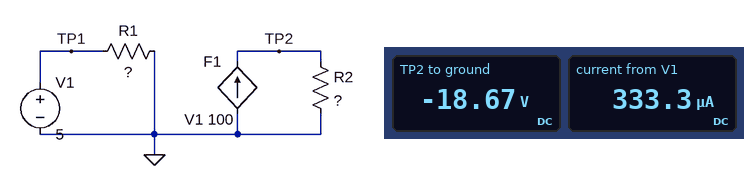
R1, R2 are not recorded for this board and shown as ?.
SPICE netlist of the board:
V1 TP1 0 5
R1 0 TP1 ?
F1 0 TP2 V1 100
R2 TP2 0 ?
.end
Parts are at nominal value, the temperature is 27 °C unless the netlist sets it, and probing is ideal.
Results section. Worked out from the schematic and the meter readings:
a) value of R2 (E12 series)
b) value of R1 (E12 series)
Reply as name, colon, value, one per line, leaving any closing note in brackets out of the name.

value of R2: 560 Ω
value of R1: 15 kΩ
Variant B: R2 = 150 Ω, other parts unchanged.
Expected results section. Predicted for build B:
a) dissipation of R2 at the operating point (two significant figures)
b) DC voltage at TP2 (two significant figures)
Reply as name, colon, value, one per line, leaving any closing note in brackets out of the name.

dissipation of R2 at the operating point: 170 mW
DC voltage at TP2: -5.0 V
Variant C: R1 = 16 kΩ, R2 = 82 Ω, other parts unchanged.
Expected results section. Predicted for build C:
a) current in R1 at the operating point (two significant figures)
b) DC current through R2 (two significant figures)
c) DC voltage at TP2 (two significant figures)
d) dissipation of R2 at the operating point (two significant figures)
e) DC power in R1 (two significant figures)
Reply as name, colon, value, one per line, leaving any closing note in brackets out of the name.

current in R1 at the operating point: 310 µA
DC current through R2: 31 mA
DC voltage at TP2: -2.6 V
dissipation of R2 at the operating point: 80 mW
DC power in R1: 1.6 mW
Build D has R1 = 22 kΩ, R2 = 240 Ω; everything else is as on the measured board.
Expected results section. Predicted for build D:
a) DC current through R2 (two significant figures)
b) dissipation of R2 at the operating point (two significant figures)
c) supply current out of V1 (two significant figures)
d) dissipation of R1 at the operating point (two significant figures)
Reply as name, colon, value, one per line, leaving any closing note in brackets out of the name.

DC current through R2: 23 mA
dissipation of R2 at the operating point: 120 mW
supply current out of V1: 230 µA
dissipation of R1 at the operating point: 1.1 mW
